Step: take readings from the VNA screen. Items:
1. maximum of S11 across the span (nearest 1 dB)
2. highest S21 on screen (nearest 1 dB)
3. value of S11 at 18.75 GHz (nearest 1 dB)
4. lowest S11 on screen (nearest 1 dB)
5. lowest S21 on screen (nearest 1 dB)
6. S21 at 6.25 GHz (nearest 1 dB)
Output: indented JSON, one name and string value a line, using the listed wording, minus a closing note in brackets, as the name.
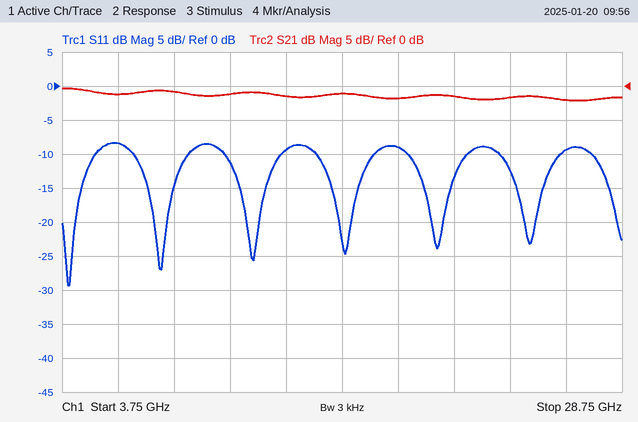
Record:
{
  "maximum of S11 across the span": "-8 dB",
  "highest S21 on screen": "0 dB",
  "value of S11 at 18.75 GHz": "-9 dB",
  "lowest S11 on screen": "-29 dB",
  "lowest S21 on screen": "-2 dB",
  "S21 at 6.25 GHz": "-1 dB"
}
